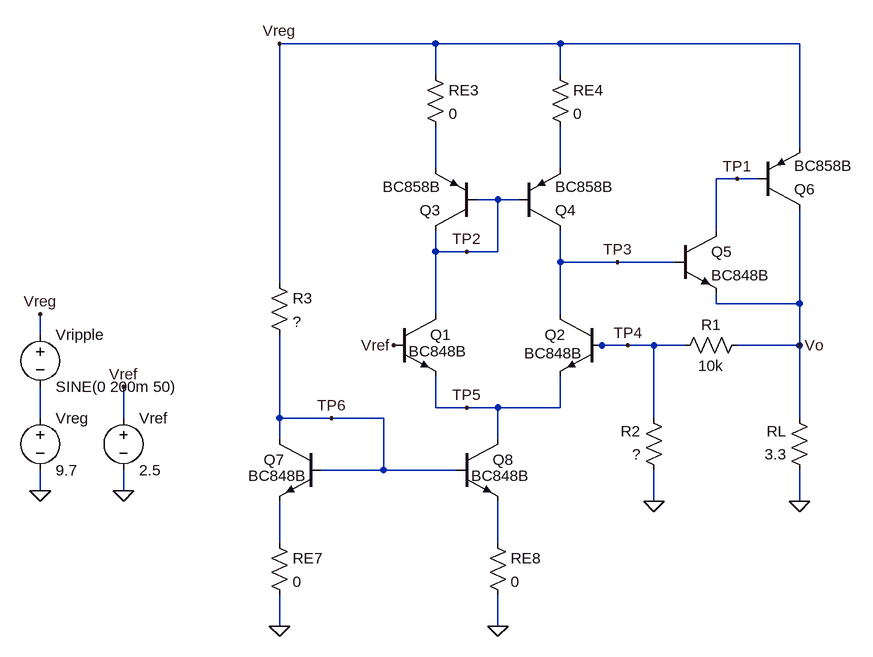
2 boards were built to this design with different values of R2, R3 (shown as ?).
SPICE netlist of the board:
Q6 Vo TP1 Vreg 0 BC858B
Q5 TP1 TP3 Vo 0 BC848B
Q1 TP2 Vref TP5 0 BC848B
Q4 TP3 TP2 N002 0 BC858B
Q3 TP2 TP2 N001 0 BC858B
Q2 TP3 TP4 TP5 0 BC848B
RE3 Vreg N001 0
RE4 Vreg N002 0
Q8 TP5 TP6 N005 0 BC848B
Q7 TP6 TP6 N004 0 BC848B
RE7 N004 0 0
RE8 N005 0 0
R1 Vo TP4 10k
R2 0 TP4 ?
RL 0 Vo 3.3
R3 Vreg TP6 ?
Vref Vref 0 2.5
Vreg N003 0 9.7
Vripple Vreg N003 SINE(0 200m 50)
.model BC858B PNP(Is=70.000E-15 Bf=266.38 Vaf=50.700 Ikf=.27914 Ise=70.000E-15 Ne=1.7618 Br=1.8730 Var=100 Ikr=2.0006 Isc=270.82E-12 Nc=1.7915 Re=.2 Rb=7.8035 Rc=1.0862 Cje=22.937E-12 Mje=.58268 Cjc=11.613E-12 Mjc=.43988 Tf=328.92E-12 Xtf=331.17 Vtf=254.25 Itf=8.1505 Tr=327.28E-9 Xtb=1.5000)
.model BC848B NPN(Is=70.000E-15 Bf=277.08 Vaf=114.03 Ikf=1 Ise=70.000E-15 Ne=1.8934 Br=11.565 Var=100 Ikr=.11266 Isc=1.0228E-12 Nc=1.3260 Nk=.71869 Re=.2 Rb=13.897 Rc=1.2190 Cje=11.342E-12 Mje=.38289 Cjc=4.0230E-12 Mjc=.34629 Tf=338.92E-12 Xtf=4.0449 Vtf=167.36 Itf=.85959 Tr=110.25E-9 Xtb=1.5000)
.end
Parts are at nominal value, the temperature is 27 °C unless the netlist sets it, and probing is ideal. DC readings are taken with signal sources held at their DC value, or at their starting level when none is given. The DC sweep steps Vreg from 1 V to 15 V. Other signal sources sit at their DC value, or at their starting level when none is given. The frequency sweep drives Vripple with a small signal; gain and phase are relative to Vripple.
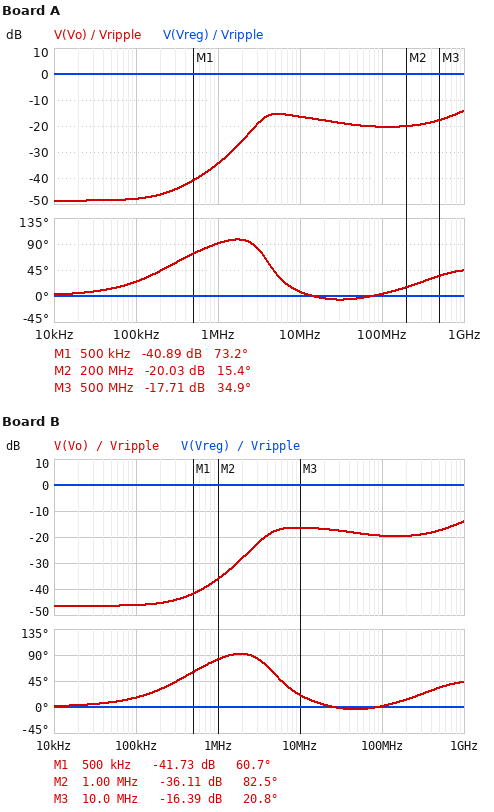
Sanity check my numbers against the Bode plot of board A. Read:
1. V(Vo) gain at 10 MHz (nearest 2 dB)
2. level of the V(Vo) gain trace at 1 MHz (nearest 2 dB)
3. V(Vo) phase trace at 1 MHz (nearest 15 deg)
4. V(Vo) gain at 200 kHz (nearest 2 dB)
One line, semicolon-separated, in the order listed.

-16 dB; -34 dB; 90 deg; -46 dB
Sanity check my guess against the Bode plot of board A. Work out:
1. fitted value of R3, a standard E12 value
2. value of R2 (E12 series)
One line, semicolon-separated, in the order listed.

12 kΩ; 22 kΩ
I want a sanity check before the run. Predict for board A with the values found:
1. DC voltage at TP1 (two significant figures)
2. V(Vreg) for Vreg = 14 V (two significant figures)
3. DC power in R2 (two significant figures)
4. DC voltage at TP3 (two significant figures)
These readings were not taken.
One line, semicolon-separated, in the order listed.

8.5 V; 14 V; 280 µW; 4.3 V
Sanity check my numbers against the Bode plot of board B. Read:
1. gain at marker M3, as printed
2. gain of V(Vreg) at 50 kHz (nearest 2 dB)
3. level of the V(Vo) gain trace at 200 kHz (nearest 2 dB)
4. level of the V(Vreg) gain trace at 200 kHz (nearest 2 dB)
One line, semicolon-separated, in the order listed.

-16.39 dB; 0 dB; -46 dB; 0 dB
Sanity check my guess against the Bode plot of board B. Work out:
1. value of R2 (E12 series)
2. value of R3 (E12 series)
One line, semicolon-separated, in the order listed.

18 kΩ; 6.8 kΩ
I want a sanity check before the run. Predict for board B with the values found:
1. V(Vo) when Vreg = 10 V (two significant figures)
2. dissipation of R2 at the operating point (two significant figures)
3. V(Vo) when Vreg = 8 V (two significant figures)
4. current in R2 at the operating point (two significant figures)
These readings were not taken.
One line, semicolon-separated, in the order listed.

3.9 V; 350 µW; 3.9 V; 140 µA
